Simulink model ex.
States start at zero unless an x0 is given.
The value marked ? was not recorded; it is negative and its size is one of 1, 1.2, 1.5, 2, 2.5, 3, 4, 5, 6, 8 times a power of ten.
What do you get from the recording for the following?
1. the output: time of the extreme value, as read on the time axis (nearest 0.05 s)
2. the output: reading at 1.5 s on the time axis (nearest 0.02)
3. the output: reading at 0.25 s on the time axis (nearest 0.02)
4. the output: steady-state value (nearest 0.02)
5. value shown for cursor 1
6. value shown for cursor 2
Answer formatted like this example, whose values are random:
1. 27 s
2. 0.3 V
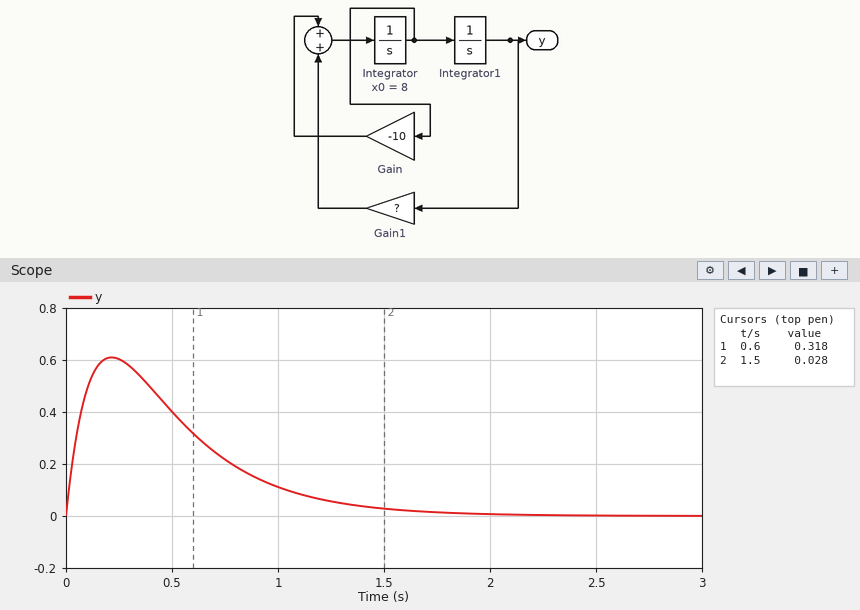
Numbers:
1. 0.20 s
2. 0.02
3. 0.60
4. 0.00
5. 0.318
6. 0.028
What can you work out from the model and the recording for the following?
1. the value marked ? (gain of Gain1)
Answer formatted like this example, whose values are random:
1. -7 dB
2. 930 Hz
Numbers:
1. -20
